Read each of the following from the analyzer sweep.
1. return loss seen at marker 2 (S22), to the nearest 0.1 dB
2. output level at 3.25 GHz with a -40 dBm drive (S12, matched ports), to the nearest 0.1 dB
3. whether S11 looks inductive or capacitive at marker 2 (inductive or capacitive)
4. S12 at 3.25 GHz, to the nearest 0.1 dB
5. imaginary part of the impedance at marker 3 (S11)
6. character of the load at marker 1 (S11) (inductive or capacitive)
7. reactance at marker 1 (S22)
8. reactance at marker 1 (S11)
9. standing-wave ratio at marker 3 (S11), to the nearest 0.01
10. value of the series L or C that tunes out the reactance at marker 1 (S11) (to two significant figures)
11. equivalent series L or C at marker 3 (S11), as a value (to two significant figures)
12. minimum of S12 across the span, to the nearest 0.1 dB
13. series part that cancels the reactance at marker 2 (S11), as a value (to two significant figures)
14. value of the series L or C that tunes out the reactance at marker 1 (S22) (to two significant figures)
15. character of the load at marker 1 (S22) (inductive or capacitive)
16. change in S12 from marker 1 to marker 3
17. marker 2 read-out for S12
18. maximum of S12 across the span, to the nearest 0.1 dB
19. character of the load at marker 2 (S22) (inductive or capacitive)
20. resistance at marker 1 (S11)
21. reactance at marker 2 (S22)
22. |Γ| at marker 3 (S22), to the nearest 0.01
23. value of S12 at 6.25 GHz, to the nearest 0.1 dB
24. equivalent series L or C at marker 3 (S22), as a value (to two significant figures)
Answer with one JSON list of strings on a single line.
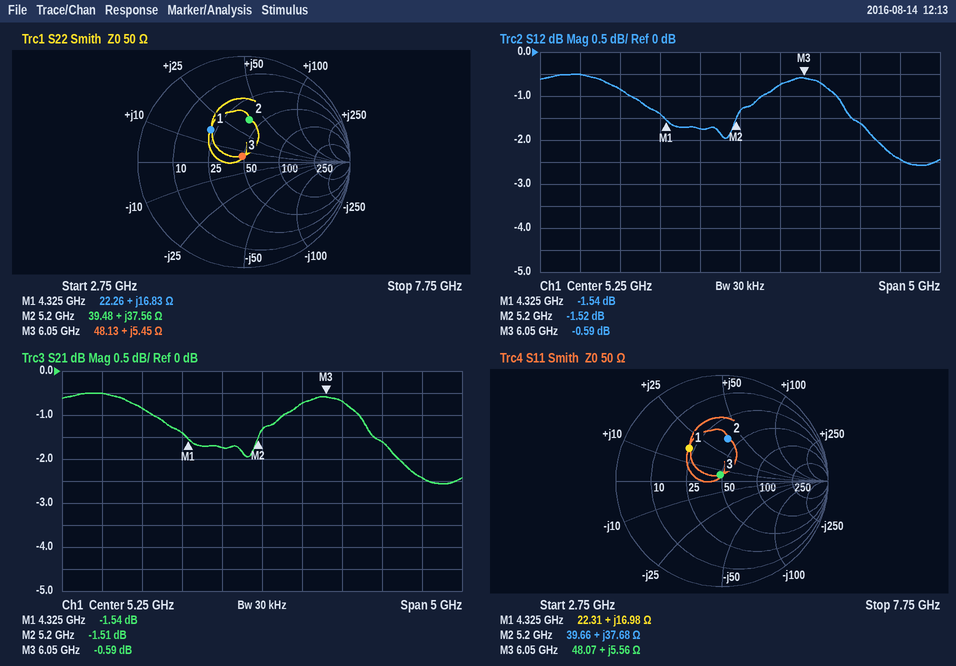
["7.9 dB", "-40.5 dBm", "inductive", "-0.5 dB", "+5.56 Ω", "inductive", "+16.83 Ω", "+16.98 Ω", "1.13", "2.2 pF", "150 pH", "-2.6 dB", "810 fF", "2.2 pF", "inductive", "0.95 dB", "-1.52 dB", "-0.5 dB", "inductive", "22.31 Ω", "+37.56 Ω", "0.06", "-0.7 dB", "140 pH"]
